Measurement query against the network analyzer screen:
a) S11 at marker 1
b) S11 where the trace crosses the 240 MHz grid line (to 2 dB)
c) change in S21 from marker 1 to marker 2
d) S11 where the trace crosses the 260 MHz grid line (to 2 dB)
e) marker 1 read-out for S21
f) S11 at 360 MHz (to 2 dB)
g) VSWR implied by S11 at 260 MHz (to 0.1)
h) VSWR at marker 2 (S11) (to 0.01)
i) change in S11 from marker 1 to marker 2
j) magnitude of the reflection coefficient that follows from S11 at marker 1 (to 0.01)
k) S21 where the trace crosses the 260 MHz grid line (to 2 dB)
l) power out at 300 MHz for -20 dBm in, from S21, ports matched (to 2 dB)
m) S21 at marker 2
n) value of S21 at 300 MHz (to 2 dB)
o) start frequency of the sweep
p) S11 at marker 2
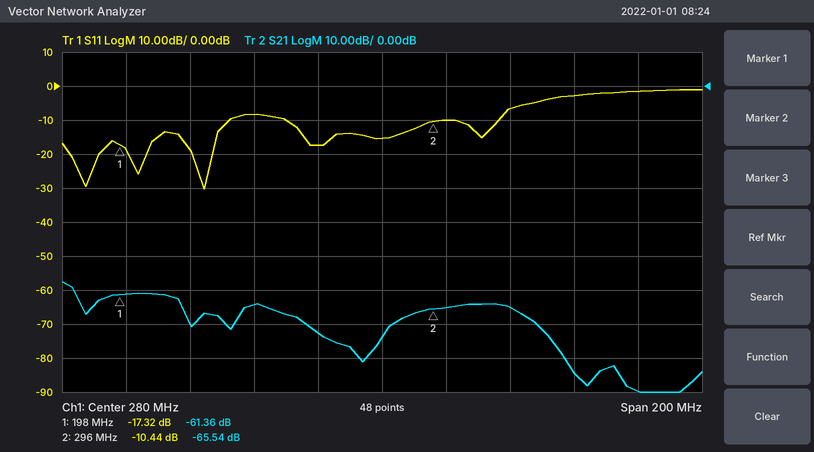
-17.32 dB
-8 dB
-4.18 dB
-18 dB
-61.36 dB
-2 dB
1.3
1.86
6.88 dB
0.14
-72 dB
-86 dBm
-65.54 dB
-66 dB
180 MHz
-10.44 dB
